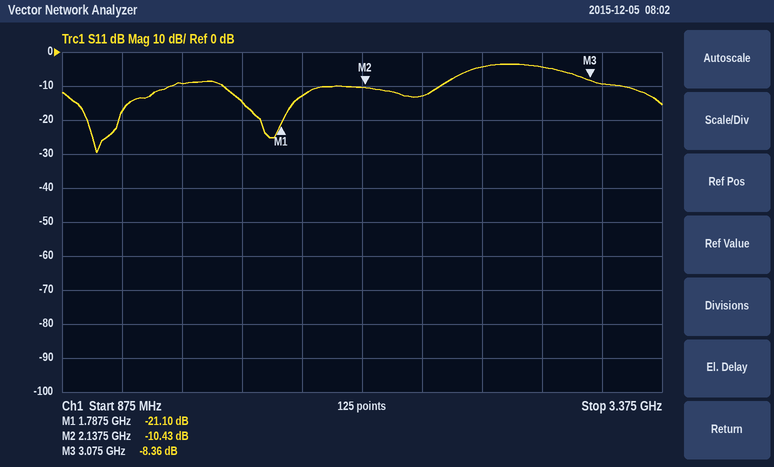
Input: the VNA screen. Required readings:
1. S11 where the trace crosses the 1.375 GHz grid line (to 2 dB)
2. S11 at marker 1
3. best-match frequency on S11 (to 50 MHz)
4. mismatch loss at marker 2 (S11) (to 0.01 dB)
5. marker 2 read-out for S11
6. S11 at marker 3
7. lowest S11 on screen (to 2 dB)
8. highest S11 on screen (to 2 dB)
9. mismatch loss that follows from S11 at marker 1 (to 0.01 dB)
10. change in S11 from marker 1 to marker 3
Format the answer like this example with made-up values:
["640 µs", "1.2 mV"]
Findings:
["-10 dB", "-21.10 dB", "1.00 GHz", "0.41 dB", "-10.43 dB", "-8.36 dB", "-30 dB", "-4 dB", "0.03 dB", "12.74 dB"]
